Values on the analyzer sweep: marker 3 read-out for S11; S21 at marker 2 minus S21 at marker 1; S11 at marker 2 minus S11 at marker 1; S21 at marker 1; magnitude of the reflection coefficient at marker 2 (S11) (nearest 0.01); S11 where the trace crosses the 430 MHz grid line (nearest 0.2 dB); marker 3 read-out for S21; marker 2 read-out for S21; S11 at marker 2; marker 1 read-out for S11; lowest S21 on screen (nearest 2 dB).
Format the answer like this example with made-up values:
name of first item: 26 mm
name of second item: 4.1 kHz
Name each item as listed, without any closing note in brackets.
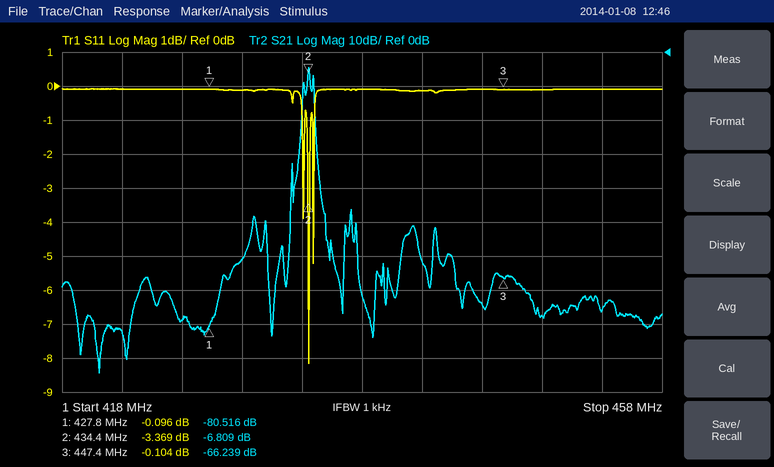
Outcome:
marker 3 read-out for S11: -0.104 dB
S21 at marker 2 minus S21 at marker 1: 73.707 dB
S11 at marker 2 minus S11 at marker 1: -3.273 dB
S21 at marker 1: -80.516 dB
magnitude of the reflection coefficient at marker 2 (S11): 0.68
S11 where the trace crosses the 430 MHz grid line: -0.2 dB
marker 3 read-out for S21: -66.239 dB
marker 2 read-out for S21: -6.809 dB
S11 at marker 2: -3.369 dB
marker 1 read-out for S11: -0.096 dB
lowest S21 on screen: -94 dB
